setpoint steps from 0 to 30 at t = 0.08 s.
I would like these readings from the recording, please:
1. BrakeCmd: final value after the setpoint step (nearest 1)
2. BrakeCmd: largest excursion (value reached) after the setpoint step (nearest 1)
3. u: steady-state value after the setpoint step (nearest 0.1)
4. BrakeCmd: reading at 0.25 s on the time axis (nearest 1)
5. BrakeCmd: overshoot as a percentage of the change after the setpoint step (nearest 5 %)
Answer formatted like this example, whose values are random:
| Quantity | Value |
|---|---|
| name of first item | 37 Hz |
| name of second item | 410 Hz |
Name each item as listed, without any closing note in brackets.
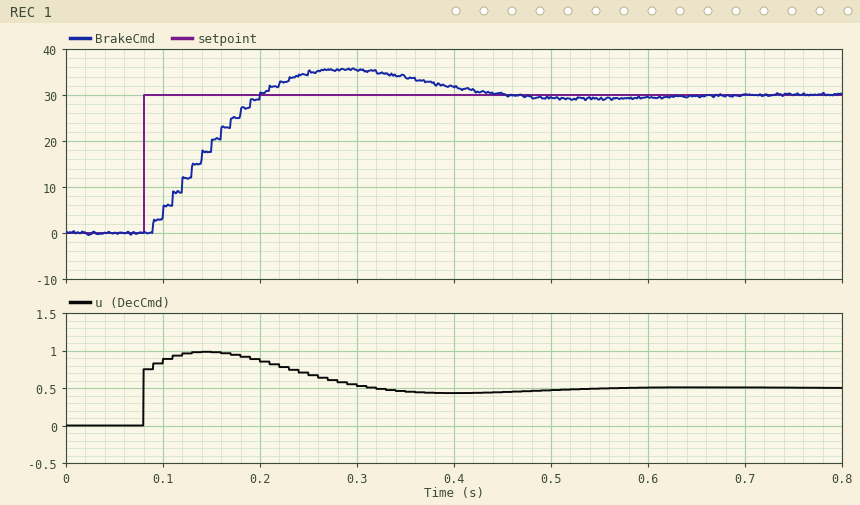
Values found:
| Quantity | Value |
|---|---|
| BrakeCmd: final value after the setpoint step | 30 |
| BrakeCmd: largest excursion (value reached) after the setpoint step | 36 |
| u: steady-state value after the setpoint step | 0.5 |
| BrakeCmd: reading at 0.25 s on the time axis | 35 |
| BrakeCmd: overshoot as a percentage of the change after the setpoint step | 20 % |
